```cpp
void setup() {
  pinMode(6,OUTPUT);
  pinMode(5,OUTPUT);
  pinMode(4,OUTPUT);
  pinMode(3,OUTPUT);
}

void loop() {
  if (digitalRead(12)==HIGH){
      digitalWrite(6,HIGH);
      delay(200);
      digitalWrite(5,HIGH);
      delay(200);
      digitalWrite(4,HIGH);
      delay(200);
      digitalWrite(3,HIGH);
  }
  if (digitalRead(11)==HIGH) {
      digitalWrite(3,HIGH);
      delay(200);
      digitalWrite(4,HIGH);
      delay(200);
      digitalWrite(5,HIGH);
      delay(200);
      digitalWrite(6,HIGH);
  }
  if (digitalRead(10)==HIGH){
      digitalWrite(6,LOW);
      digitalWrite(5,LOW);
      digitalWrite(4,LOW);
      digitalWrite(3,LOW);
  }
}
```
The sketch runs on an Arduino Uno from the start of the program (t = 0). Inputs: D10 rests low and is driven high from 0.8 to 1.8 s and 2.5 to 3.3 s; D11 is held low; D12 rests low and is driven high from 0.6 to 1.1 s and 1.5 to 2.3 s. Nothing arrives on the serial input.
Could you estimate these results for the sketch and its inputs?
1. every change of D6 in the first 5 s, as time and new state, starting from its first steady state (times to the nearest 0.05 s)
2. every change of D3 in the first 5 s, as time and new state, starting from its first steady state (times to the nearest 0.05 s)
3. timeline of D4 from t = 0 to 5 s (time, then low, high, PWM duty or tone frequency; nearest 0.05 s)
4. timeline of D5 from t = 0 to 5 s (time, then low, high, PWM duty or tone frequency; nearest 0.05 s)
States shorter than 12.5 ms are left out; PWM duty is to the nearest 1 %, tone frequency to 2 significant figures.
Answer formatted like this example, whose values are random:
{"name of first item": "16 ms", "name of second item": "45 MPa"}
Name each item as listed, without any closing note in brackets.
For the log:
{"every change of D6 in the first 5 s, as time and new state, starting from its first steady state": "0 s low; 0.6 s high; 1.2 s low; 1.5 s high; 2.7 s low", "every change of D3 in the first 5 s, as time and new state, starting from its first steady state": "0 s low; 2.1 s high; 2.7 s low", "timeline of D4 from t = 0 to 5 s": "0 s low; 1 s high; 1.2 s low; 1.9 s high; 2.7 s low", "timeline of D5 from t = 0 to 5 s": "0 s low; 0.8 s high; 1.2 s low; 1.7 s high; 2.7 s low"}
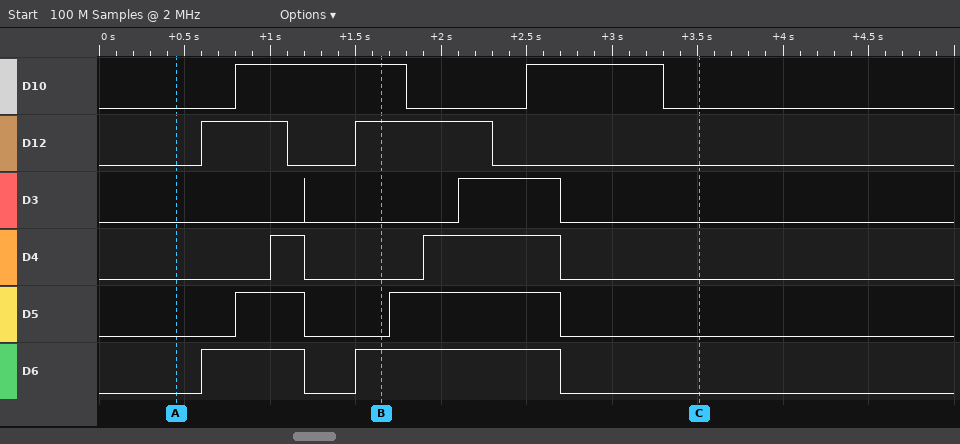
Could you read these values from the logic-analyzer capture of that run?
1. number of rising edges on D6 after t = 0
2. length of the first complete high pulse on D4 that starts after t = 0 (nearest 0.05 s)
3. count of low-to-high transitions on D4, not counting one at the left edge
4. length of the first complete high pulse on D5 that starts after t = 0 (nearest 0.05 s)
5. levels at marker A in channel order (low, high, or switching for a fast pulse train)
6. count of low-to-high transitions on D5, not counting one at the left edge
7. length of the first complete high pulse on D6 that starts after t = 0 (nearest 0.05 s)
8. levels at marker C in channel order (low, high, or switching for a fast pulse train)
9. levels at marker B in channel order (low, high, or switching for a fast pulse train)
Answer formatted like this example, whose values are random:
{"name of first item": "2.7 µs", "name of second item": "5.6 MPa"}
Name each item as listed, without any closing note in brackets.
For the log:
{"number of rising edges on D6 after t = 0": "2", "length of the first complete high pulse on D4 that starts after t = 0": "0.20 s", "count of low-to-high transitions on D4, not counting one at the left edge": "2", "length of the first complete high pulse on D5 that starts after t = 0": "0.40 s", "levels at marker A in channel order": "D10 low, D12 low, D3 low, D4 low, D5 low, D6 low", "count of low-to-high transitions on D5, not counting one at the left edge": "2", "length of the first complete high pulse on D6 that starts after t = 0": "0.60 s", "levels at marker C in channel order": "D10 low, D12 low, D3 low, D4 low, D5 low, D6 low", "levels at marker B in channel order": "D10 high, D12 high, D3 low, D4 low, D5 low, D6 high"}
